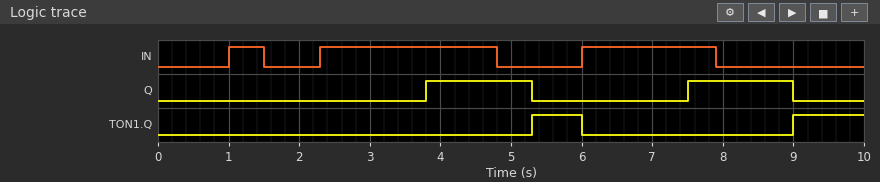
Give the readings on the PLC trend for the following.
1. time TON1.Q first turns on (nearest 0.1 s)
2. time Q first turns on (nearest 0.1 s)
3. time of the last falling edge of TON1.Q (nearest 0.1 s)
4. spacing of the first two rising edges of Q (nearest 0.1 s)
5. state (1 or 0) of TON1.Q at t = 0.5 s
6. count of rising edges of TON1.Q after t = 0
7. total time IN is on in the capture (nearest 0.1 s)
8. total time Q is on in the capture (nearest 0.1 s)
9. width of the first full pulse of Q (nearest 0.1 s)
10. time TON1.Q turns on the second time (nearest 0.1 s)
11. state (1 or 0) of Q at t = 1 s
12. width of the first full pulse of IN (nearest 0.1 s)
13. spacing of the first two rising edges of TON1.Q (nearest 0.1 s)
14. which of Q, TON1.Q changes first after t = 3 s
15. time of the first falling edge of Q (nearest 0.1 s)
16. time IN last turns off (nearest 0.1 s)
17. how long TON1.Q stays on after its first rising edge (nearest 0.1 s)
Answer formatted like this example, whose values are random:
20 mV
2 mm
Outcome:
5.3 s
3.8 s
6.0 s
3.7 s
0
2
4.9 s
3.0 s
1.5 s
9.0 s
0
0.5 s
3.7 s
Q
5.3 s
7.9 s
0.7 s
